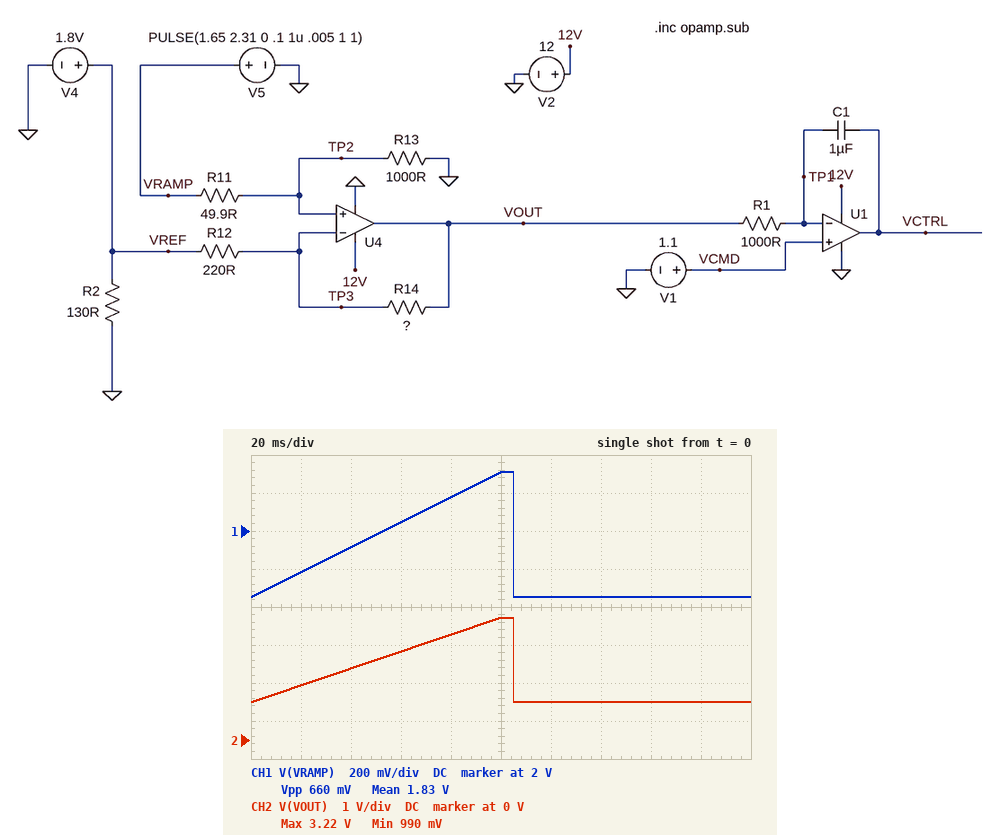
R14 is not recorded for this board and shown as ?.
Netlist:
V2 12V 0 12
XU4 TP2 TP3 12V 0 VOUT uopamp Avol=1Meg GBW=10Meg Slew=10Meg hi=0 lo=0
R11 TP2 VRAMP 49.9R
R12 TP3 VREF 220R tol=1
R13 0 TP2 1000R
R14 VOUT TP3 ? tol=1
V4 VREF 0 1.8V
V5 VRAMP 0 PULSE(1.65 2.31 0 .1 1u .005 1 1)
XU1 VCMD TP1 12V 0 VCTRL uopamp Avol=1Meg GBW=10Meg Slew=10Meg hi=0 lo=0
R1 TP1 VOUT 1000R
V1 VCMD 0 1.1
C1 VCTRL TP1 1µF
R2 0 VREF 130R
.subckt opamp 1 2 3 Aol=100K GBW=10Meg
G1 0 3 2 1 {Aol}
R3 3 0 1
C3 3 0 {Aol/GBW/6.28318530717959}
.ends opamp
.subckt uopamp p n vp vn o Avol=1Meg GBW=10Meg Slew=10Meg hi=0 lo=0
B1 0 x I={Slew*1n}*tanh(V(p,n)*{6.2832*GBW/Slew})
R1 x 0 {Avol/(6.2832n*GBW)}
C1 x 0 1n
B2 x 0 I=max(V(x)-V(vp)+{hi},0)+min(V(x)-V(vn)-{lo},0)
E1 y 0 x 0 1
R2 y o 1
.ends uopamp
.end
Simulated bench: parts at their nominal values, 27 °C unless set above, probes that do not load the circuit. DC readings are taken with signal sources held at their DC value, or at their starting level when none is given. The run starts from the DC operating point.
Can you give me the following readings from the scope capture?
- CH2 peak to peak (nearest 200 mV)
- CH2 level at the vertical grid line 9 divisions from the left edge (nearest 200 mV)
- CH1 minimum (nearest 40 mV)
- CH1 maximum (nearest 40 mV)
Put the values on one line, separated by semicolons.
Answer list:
2.2 V; 1.0 V; 1.64 V; 2.32 V
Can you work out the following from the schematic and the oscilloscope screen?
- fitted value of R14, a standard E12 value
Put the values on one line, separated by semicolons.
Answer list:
560 Ω
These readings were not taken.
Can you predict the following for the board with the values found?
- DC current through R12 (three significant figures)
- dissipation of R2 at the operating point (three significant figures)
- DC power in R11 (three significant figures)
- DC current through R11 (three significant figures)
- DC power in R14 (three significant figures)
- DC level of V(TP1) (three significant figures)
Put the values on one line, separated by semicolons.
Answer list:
1.04 mA; 24.9 mW; 123 µW; 1.57 mA; 604 µW; 990 mV
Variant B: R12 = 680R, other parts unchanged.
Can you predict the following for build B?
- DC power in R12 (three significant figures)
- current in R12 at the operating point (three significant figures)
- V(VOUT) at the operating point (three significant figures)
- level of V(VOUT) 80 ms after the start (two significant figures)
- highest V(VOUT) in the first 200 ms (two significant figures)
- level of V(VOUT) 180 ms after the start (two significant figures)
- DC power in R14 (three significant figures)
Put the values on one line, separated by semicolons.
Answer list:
76.7 µW; 336 µA; 1.38 V; 2.3 V; 2.5 V; 1.4 V; 63.2 µW
